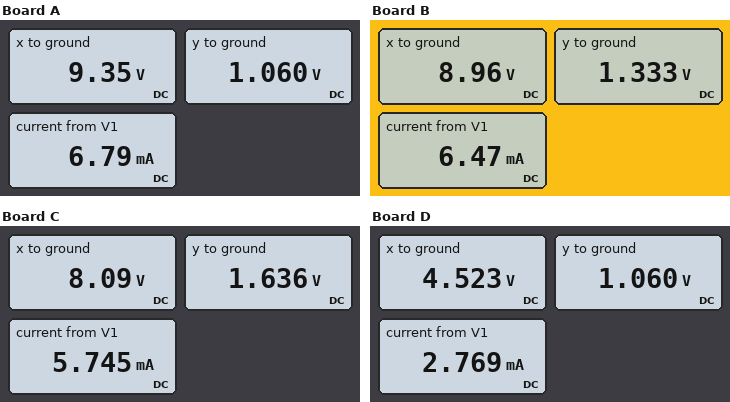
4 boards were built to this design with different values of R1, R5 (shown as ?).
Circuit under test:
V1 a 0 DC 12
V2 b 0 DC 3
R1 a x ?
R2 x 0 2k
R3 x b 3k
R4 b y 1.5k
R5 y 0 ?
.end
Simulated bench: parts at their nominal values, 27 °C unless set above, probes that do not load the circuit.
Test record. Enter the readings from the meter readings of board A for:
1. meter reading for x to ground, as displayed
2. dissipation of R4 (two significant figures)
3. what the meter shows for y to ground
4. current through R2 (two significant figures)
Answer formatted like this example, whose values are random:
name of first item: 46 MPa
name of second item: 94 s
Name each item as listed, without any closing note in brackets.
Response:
meter reading for x to ground, as displayed: 9.35 V
dissipation of R4: 2.5 mW
what the meter shows for y to ground: 1.060 V
current through R2: 4.7 mA
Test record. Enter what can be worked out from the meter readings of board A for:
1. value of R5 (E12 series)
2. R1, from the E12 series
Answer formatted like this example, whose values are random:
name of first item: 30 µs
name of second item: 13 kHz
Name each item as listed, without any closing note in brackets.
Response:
value of R5: 820 Ω
R1, from the E12 series: 390 Ω
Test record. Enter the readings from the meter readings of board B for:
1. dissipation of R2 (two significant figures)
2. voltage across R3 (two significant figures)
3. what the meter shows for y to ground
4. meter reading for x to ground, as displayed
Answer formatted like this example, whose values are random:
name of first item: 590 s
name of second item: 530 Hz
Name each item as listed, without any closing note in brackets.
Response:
dissipation of R2: 40 mW
voltage across R3: 6.0 V
what the meter shows for y to ground: 1.333 V
meter reading for x to ground, as displayed: 8.96 V
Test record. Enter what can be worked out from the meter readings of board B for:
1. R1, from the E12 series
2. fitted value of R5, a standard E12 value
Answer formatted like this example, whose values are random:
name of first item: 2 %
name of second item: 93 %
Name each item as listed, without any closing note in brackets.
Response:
R1, from the E12 series: 470 Ω
fitted value of R5, a standard E12 value: 1.2 kΩ
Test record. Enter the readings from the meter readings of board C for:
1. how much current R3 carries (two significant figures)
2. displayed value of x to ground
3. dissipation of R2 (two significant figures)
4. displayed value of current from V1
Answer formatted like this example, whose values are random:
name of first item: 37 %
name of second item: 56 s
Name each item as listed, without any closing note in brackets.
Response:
how much current R3 carries: 1.7 mA
displayed value of x to ground: 8.09 V
dissipation of R2: 33 mW
displayed value of current from V1: 5.745 mA
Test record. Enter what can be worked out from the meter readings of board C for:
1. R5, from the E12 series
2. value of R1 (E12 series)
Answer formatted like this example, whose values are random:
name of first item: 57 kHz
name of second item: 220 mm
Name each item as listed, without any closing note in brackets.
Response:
R5, from the E12 series: 1.8 kΩ
value of R1: 680 Ω
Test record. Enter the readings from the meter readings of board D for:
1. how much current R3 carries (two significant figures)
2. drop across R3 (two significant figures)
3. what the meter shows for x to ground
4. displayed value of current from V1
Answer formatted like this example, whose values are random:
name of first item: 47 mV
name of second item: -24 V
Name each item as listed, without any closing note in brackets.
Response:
how much current R3 carries: 510 µA
drop across R3: 1.5 V
what the meter shows for x to ground: 4.523 V
displayed value of current from V1: 2.769 mA
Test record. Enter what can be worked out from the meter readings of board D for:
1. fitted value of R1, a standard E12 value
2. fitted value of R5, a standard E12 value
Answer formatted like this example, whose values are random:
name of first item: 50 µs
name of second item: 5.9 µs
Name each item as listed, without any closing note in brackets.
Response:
fitted value of R1, a standard E12 value: 2.7 kΩ
fitted value of R5, a standard E12 value: 820 Ω
